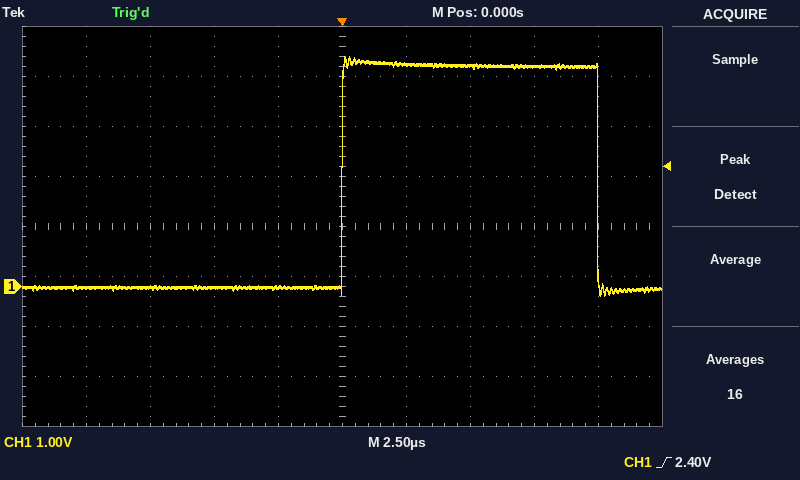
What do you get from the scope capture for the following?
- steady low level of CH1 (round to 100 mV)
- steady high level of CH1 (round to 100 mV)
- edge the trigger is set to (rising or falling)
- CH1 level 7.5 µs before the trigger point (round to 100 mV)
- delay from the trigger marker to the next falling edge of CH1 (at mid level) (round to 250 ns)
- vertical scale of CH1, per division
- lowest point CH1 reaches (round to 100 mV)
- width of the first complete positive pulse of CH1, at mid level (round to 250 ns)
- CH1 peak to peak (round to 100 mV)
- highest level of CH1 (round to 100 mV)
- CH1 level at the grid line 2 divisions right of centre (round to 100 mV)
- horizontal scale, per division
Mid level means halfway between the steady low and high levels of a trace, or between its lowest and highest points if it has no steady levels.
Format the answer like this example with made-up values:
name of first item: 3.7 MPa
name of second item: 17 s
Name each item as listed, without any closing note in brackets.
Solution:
steady low level of CH1: 0.0 V
steady high level of CH1: 4.4 V
edge the trigger is set to: rising
CH1 level 7.5 µs before the trigger point: 0.0 V
delay from the trigger marker to the next falling edge of CH1 (at mid level): 10.00 µs
vertical scale of CH1, per division: 1 V
lowest point CH1 reaches: -200 mV
width of the first complete positive pulse of CH1, at mid level: 10.00 µs
CH1 peak to peak: 4.8 V
highest level of CH1: 4.6 V
CH1 level at the grid line 2 divisions right of centre: 4.4 V
horizontal scale, per division: 2.5 µs
